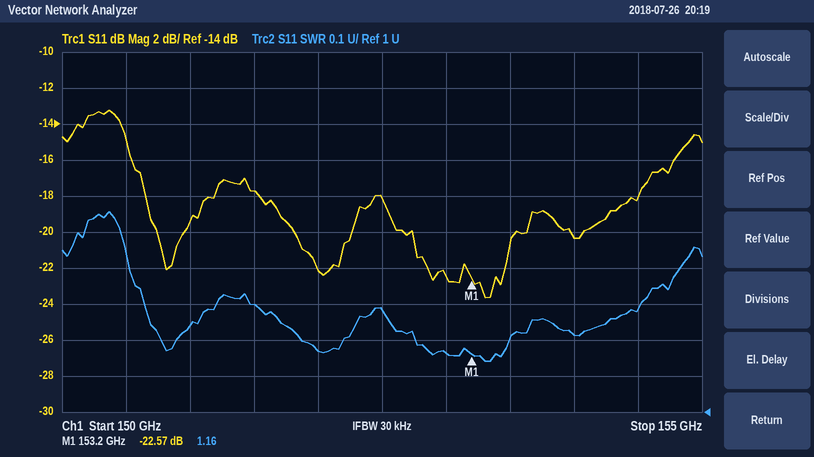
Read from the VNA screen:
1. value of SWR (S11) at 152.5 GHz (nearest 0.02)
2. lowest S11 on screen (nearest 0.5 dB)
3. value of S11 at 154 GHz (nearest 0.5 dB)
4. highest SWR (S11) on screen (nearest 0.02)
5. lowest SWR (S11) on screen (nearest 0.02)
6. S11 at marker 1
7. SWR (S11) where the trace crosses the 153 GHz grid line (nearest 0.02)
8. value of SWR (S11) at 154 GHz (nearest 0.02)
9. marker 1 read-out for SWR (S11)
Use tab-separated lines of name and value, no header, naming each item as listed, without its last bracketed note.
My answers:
value of SWR (S11) at 152.5 GHz	1.28
lowest S11 on screen	-23.5 dB
value of S11 at 154 GHz	-20.5 dB
highest SWR (S11) on screen	1.56
lowest SWR (S11) on screen	1.14
S11 at marker 1	-22.57 dB
SWR (S11) where the trace crosses the 153 GHz grid line	1.16
value of SWR (S11) at 154 GHz	1.22
marker 1 read-out for SWR	1.16
